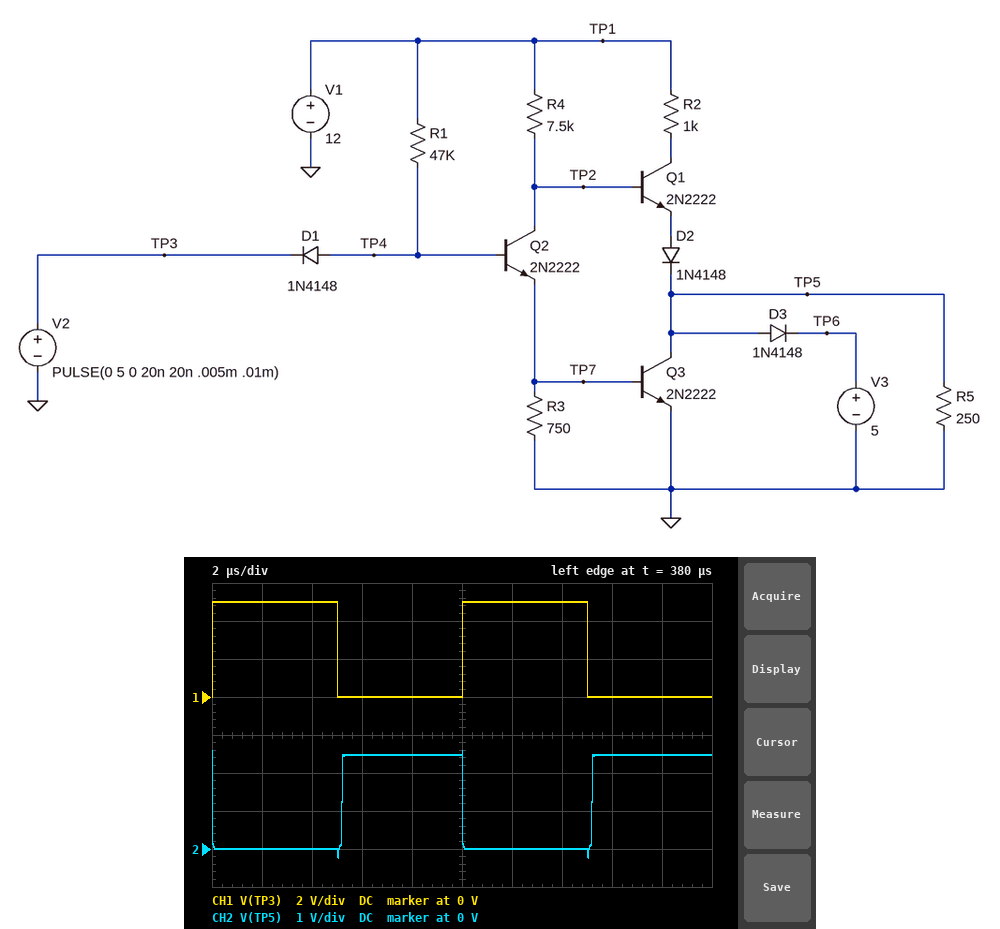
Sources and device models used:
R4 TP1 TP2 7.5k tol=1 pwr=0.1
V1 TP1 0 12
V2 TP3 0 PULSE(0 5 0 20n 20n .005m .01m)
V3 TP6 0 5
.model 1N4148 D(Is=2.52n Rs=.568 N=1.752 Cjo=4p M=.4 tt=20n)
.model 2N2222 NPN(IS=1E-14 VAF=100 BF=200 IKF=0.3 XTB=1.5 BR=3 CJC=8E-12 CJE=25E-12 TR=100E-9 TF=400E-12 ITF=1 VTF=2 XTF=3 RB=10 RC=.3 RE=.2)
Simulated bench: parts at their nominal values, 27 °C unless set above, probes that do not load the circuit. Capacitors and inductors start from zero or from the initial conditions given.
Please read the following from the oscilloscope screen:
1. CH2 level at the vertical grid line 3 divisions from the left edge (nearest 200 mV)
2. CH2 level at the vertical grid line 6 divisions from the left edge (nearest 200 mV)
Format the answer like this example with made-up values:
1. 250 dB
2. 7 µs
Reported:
1. 2.4 V
2. 0 V
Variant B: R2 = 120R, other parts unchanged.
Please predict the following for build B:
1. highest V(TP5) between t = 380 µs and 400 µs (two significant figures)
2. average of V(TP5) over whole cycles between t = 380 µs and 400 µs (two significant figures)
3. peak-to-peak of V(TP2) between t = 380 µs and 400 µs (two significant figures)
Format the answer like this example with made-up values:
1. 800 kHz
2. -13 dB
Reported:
1. 5.7 V
2. 2.8 V
3. 7.3 V
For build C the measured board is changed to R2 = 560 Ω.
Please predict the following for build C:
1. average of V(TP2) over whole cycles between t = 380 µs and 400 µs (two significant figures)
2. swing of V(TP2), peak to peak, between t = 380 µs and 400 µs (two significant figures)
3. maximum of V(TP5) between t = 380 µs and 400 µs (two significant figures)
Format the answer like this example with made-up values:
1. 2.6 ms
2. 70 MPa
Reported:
1. 2.8 V
2. 5.2 V
3. 3.7 V
